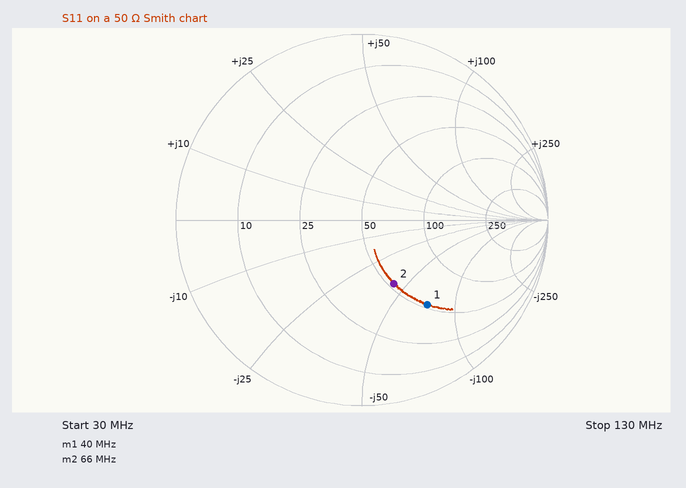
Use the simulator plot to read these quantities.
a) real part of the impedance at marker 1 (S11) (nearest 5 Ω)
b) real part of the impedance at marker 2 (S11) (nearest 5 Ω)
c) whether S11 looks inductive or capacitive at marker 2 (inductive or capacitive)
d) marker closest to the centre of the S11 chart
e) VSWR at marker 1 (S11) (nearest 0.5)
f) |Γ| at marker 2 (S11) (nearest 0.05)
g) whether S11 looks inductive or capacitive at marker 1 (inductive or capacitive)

55 Ω
55 Ω
capacitive
marker 2
3.5
0.40
capacitive
